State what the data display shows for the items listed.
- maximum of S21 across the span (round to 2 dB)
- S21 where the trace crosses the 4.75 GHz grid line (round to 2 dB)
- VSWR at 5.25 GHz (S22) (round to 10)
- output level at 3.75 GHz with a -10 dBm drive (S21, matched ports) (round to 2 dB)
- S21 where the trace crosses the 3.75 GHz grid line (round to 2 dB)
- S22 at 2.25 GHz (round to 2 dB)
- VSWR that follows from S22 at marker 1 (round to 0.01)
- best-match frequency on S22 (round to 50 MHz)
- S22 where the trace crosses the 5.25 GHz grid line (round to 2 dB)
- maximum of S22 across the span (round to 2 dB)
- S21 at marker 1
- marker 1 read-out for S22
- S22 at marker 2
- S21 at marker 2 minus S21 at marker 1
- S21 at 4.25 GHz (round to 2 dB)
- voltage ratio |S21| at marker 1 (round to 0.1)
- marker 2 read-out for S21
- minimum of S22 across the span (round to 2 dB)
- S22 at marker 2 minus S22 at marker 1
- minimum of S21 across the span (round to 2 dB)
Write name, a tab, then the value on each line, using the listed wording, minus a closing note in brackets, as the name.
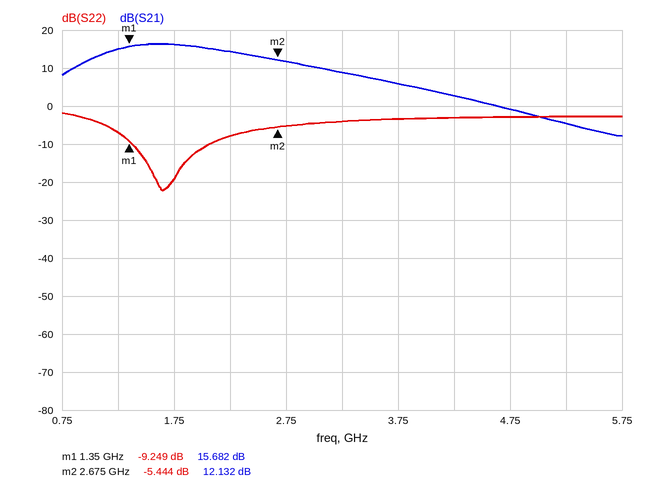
maximum of S21 across the span	16 dB
S21 where the trace crosses the 4.75 GHz grid line	0 dB
VSWR at 5.25 GHz (S22)	10
output level at 3.75 GHz with a -10 dBm drive (S21, matched ports)	-4 dBm
S21 where the trace crosses the 3.75 GHz grid line	6 dB
S22 at 2.25 GHz	-8 dB
VSWR that follows from S22 at marker 1	2.05
best-match frequency on S22	1.65 GHz
S22 where the trace crosses the 5.25 GHz grid line	-2 dB
maximum of S22 across the span	-2 dB
S21 at marker 1	15.682 dB
marker 1 read-out for S22	-9.249 dB
S22 at marker 2	-5.444 dB
S21 at marker 2 minus S21 at marker 1	-3.550 dB
S21 at 4.25 GHz	2 dB
voltage ratio |S21| at marker 1	6.1
marker 2 read-out for S21	12.132 dB
minimum of S22 across the span	-22 dB
S22 at marker 2 minus S22 at marker 1	3.805 dB
minimum of S21 across the span	-8 dB
